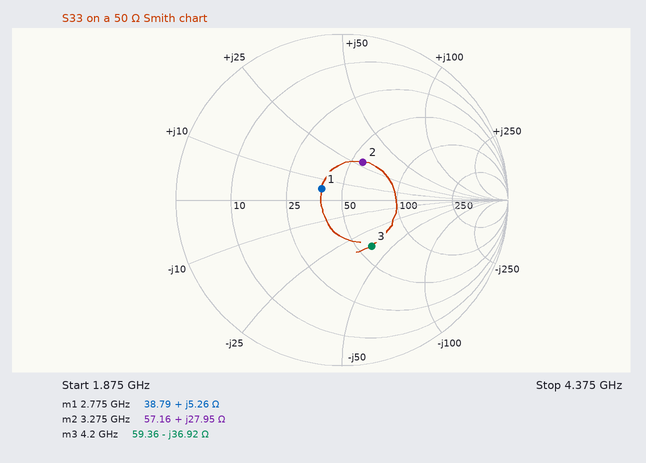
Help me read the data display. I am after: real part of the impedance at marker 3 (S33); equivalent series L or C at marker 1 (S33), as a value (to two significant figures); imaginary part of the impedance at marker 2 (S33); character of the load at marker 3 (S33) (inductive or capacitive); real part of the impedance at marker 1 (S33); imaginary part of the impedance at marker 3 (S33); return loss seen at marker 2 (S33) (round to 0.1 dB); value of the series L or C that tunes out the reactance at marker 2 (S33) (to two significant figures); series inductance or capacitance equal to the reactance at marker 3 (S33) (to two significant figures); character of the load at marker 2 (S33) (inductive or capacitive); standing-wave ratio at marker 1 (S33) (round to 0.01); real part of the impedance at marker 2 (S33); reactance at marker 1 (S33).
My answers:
59.36 Ω
300 pH
+27.95 Ω
capacitive
38.79 Ω
-36.92 Ω
11.7 dB
1.7 pF
1.0 pF
inductive
1.32
57.16 Ω
+5.26 Ω
